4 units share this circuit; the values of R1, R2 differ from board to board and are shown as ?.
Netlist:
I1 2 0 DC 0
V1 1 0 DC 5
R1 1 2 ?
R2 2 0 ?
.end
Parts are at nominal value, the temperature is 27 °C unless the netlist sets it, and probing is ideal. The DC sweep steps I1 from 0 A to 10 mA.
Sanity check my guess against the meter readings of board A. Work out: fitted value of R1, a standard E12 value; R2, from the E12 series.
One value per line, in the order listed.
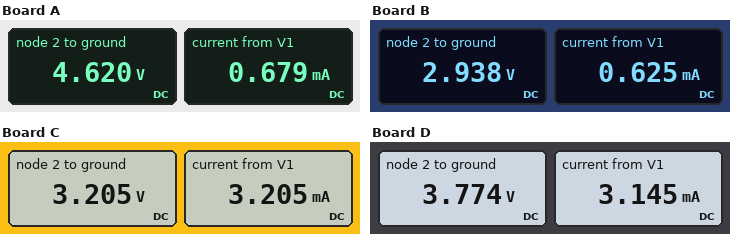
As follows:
560 Ω
6.8 kΩ
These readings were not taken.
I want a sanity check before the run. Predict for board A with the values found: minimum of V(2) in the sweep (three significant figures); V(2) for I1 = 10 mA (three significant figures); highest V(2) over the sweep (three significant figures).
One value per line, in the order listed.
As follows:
-554 mV
-554 mV
4.62 V
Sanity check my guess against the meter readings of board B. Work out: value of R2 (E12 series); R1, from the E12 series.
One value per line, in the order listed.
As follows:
4.7 kΩ
3.3 kΩ
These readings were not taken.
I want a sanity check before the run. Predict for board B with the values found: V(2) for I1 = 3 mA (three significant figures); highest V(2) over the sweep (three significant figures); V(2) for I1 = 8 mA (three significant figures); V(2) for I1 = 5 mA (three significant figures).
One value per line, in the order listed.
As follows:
-2.88 V
2.94 V
-12.6 V
-6.76 V
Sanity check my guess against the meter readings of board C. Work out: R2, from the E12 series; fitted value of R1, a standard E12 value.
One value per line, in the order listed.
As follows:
1 kΩ
560 Ω
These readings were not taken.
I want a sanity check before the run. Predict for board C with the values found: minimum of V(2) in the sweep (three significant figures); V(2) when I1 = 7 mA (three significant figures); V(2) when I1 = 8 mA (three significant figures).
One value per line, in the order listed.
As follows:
-385 mV
692 mV
333 mV
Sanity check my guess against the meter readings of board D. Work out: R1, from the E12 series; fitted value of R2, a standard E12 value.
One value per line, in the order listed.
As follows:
390 Ω
1.2 kΩ
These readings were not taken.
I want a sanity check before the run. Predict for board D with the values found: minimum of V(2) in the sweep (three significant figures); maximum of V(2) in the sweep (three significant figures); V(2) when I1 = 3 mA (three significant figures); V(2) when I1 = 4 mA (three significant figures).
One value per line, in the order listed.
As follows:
830 mV
3.77 V
2.89 V
2.60 V
